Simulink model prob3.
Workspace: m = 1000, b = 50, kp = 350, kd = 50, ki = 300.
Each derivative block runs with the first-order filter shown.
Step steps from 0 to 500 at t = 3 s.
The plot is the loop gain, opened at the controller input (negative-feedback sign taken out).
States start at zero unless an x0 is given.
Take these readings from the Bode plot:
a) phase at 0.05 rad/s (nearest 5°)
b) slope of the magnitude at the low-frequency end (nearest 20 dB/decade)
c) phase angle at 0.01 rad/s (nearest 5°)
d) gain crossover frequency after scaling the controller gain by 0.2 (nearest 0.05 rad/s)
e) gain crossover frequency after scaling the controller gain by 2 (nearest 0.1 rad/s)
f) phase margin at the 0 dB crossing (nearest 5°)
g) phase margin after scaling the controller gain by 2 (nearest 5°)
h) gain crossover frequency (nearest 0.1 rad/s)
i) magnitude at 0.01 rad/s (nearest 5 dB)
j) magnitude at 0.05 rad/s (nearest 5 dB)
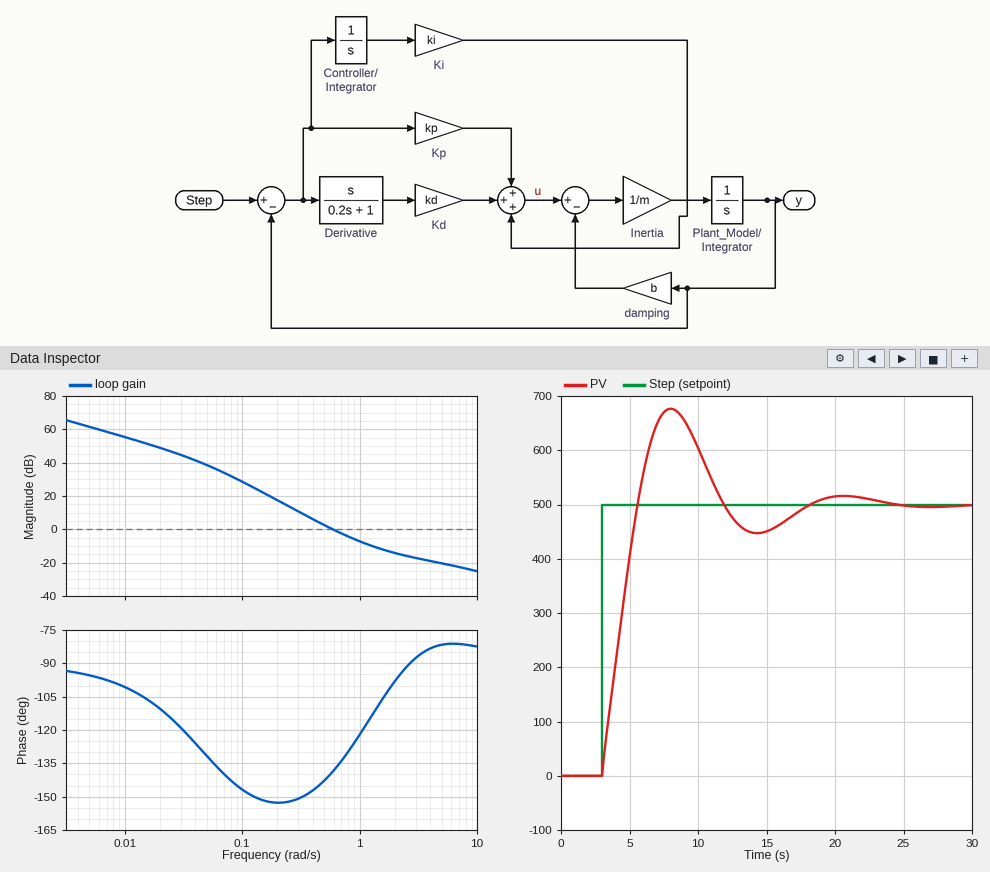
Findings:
-130°
-20 dB/decade
-100°
0.25 rad/s
0.9 rad/s
40°
55°
0.6 rad/s
55 dB
40 dB
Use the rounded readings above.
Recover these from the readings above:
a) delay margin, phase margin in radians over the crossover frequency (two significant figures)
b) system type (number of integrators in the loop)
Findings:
1.2 s
1
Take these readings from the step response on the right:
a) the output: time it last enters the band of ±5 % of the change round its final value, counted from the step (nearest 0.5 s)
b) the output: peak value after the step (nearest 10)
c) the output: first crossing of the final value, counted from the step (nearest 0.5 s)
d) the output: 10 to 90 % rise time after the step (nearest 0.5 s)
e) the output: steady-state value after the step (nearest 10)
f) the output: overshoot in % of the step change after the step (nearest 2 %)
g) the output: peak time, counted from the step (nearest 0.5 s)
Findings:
13.5 s
680
2.5 s
2.0 s
500
36 %
5.0 s
